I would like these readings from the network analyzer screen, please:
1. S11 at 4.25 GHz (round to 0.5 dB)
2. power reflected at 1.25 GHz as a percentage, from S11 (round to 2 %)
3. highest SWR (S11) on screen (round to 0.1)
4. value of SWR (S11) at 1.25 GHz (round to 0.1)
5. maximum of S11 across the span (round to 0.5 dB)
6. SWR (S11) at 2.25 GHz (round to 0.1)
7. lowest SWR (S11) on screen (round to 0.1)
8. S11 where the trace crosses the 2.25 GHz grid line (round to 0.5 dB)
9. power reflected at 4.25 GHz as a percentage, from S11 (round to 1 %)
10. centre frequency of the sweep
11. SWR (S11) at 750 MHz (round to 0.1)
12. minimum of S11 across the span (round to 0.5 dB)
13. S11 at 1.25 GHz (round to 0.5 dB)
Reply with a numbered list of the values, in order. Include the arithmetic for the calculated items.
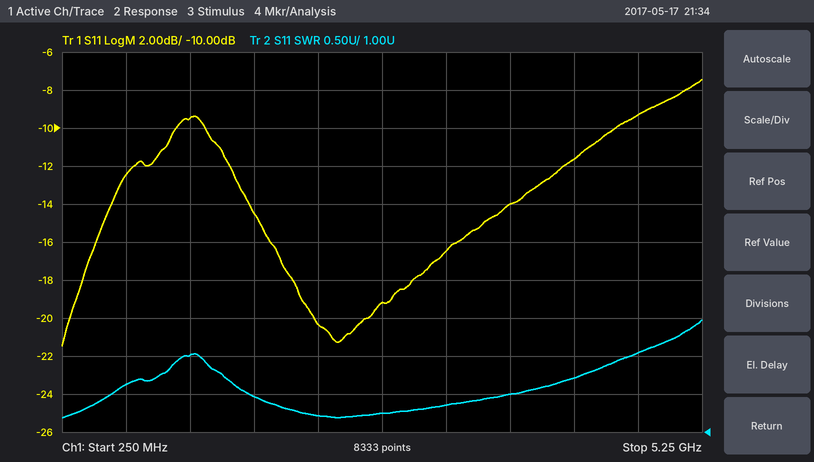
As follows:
1. -11.5 dB
2. 10^(-9.5/10) ≈ 11.2 %, so 12 % to the nearest 2 %
3. 2.5
4. 2.0
5. -7.5 dB
6. 1.2
7. 1.2
8. -20.5 dB
9. 10^(-11.5/10) ≈ 7 %
10. 2.75 GHz
11. 1.6
12. -21.5 dB
13. -9.5 dB
